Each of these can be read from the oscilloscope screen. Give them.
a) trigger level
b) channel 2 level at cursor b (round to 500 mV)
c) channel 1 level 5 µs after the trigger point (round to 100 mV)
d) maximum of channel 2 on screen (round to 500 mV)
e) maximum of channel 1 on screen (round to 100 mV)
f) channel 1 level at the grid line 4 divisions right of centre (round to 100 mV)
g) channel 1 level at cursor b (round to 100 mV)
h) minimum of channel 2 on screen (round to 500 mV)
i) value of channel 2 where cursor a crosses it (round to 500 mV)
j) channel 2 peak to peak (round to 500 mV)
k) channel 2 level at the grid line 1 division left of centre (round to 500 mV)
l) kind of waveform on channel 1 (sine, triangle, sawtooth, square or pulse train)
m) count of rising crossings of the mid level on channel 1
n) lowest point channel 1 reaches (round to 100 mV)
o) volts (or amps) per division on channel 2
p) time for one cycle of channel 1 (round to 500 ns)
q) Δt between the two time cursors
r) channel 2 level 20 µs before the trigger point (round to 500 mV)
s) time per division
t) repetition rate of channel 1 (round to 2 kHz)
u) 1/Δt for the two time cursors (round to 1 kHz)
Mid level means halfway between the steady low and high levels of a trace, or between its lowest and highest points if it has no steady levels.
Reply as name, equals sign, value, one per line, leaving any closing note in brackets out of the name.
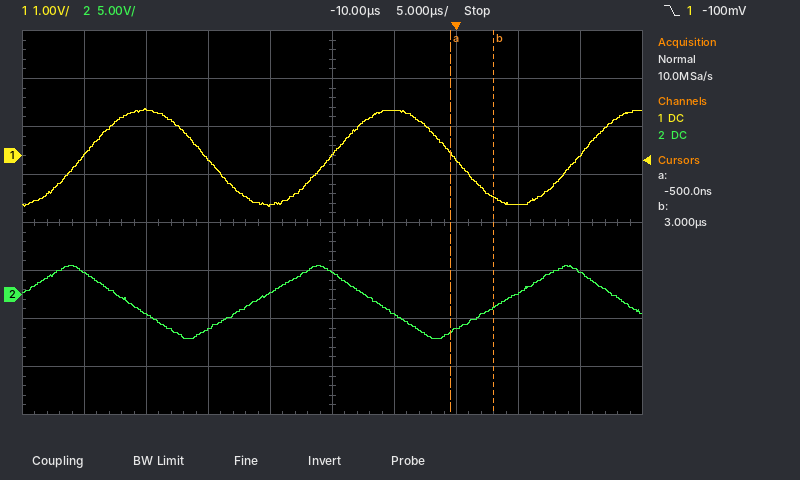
trigger level = -100 mV
channel 2 level at cursor b = -1.5 V
channel 1 level 5 µs after the trigger point = -1.0 V
maximum of channel 2 on screen = 3.0 V
maximum of channel 1 on screen = 1.0 V
channel 1 level at the grid line 4 divisions right of centre = 0.0 V
channel 1 level at cursor b = -900 mV
minimum of channel 2 on screen = -4.5 V
value of channel 2 where cursor a crosses it = -4.0 V
channel 2 peak to peak = 7.5 V
channel 2 level at the grid line 1 division left of centre = 0.0 V
kind of waveform on channel 1 = sine
count of rising crossings of the mid level on channel 1 = 3
lowest point channel 1 reaches = -1.1 V
volts (or amps) per division on channel 2 = 5 V
time for one cycle of channel 1 = 20.0 µs
Δt between the two time cursors = 3.5 µs
channel 2 level 20 µs before the trigger point = -3.5 V
time per division = 5 µs
repetition rate of channel 1 = 50 kHz
1/Δt for the two time cursors = 286 kHz
